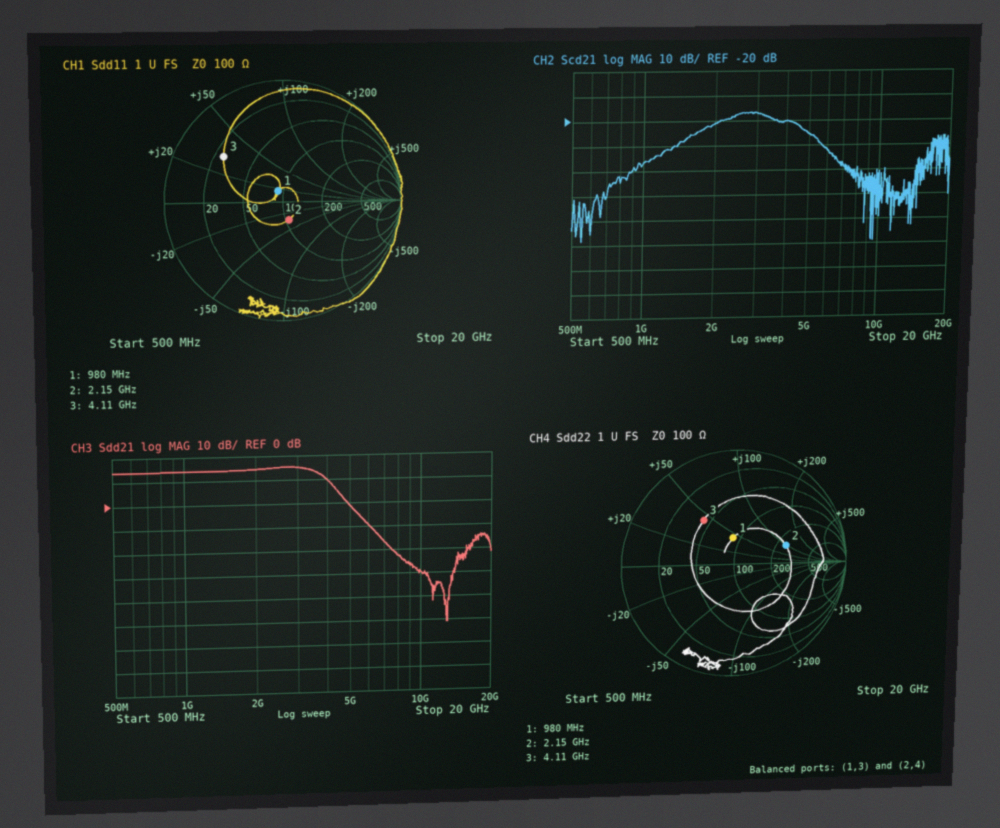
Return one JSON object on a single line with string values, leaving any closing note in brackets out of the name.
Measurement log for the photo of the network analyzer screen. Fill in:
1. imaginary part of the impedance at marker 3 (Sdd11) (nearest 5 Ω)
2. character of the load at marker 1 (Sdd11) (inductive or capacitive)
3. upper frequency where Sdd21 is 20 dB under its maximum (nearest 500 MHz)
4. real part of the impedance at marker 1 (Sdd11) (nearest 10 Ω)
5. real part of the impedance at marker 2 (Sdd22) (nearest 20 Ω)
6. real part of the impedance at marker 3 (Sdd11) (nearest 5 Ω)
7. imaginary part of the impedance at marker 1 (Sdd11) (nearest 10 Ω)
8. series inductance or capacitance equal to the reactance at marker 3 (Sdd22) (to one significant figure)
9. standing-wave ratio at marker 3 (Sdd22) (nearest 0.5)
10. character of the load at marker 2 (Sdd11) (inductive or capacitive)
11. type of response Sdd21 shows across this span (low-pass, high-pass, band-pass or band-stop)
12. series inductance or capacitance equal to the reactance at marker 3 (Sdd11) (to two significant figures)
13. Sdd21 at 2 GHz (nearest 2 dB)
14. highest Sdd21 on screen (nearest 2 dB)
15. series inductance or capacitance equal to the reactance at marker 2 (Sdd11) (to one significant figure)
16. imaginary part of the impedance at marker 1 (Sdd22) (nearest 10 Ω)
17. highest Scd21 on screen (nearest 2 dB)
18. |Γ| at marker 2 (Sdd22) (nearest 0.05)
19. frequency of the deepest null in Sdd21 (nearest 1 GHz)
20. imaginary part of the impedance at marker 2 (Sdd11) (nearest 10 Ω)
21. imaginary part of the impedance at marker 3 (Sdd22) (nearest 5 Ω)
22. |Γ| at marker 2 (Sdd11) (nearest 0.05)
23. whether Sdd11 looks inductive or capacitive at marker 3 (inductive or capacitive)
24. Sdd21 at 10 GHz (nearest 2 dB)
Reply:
{"imaginary part of the impedance at marker 3 (Sdd11)": "+30 Ω", "character of the load at marker 1 (Sdd11)": "inductive", "upper frequency where Sdd21 is 20 dB under its maximum": "5.5 GHz", "real part of the impedance at marker 1 (Sdd11)": "90 Ω", "real part of the impedance at marker 2 (Sdd22)": "240 Ω", "real part of the impedance at marker 3 (Sdd11)": "25 Ω", "imaginary part of the impedance at marker 1 (Sdd11)": "+20 Ω", "series inductance or capacitance equal to the reactance at marker 3 (Sdd22)": "2 nH", "standing-wave ratio at marker 3 (Sdd22)": "3.0", "character of the load at marker 2 (Sdd11)": "capacitive", "type of response Sdd21 shows across this span": "low-pass", "series inductance or capacitance equal to the reactance at marker 3 (Sdd11)": "1.2 nH", "Sdd21 at 2 GHz": "14 dB", "highest Sdd21 on screen": "16 dB", "series inductance or capacitance equal to the reactance at marker 2 (Sdd11)": "2 pF", "imaginary part of the impedance at marker 1 (Sdd22)": "+40 Ω", "highest Scd21 on screen": "-16 dB", "|Γ| at marker 2 (Sdd22)": "0.50", "frequency of the deepest null in Sdd21": "13 GHz", "imaginary part of the impedance at marker 2 (Sdd11)": "-30 Ω", "imaginary part of the impedance at marker 3 (Sdd22)": "+45 Ω", "|Γ| at marker 2 (Sdd11)": "0.15", "whether Sdd11 looks inductive or capacitive at marker 3": "inductive", "Sdd21 at 10 GHz": "-30 dB"}
